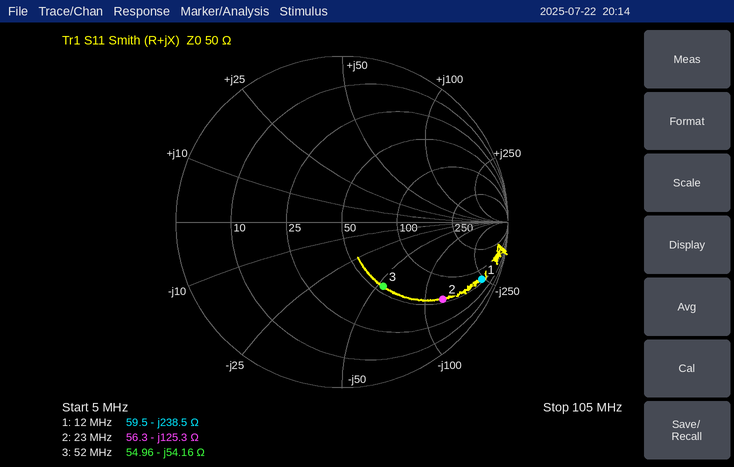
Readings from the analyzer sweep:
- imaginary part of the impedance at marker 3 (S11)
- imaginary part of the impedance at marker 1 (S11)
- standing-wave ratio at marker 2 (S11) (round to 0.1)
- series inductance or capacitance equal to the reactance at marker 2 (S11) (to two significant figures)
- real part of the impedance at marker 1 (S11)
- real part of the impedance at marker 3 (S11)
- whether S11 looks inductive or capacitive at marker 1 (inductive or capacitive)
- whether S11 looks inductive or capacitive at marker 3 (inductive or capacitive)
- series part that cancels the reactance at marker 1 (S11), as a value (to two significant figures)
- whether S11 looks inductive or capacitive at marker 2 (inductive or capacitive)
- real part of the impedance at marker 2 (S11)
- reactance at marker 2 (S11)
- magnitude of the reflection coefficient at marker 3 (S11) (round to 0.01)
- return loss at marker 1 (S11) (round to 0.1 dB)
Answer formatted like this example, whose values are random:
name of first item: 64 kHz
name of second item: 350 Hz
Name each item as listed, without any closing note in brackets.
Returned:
imaginary part of the impedance at marker 3: -54.16 Ω
imaginary part of the impedance at marker 1: -238.5 Ω
standing-wave ratio at marker 2 (S11): 7.5
series inductance or capacitance equal to the reactance at marker 2 (S11): 55 pF
real part of the impedance at marker 1: 59.5 Ω
real part of the impedance at marker 3: 54.96 Ω
whether S11 looks inductive or capacitive at marker 1: capacitive
whether S11 looks inductive or capacitive at marker 3: capacitive
series part that cancels the reactance at marker 1 (S11), as a value: 3.2 µH
whether S11 looks inductive or capacitive at marker 2: capacitive
real part of the impedance at marker 2: 56.3 Ω
reactance at marker 2: -125.3 Ω
magnitude of the reflection coefficient at marker 3 (S11): 0.46
return loss at marker 1 (S11): 0.8 dB
